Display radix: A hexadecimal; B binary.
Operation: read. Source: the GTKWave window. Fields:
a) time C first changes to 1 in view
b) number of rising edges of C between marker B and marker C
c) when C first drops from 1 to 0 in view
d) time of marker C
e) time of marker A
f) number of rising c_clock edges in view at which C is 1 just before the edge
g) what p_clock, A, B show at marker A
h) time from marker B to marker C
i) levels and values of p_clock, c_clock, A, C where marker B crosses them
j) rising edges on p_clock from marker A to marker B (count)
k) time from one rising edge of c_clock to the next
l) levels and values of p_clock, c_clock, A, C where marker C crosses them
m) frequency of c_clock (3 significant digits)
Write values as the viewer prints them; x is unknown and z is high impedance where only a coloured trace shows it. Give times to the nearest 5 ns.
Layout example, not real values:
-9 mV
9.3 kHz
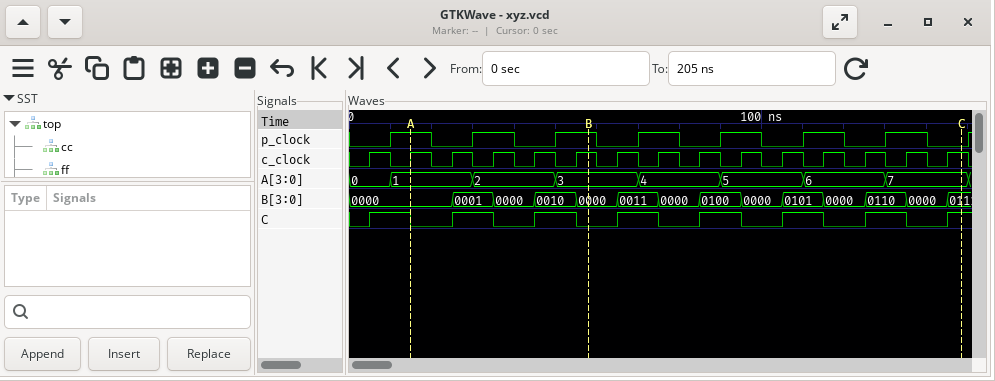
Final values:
5 ns
5
15 ns
150 ns
15 ns
7
p_clock=1, A=1, B=0000
90 ns
p_clock=1, c_clock=1, A=3, C=0
2
10 ns
p_clock=0, c_clock=1, A=7, C=1
100 MHz
